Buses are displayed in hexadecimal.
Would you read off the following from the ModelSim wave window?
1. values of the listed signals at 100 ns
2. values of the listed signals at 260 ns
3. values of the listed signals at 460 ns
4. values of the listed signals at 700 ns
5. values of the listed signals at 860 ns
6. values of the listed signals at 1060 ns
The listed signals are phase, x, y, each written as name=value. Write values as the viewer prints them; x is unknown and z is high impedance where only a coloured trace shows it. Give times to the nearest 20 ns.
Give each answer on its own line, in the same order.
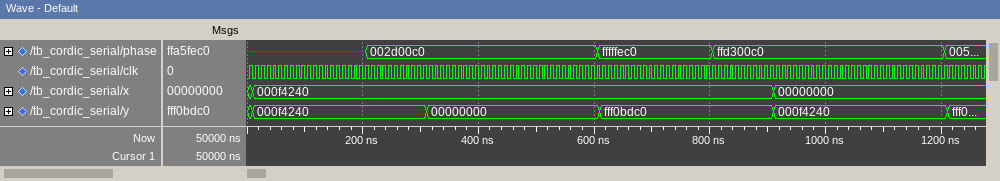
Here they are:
phase=x, x=000f4240, y=000f4240
phase=002d00c0, x=000f4240, y=000f4240
phase=002d00c0, x=000f4240, y=00000000
phase=fffffec0, x=000f4240, y=fff0bdc0
phase=ffd300c0, x=000f4240, y=fff0bdc0
phase=ffd300c0, x=00000000, y=000f4240
